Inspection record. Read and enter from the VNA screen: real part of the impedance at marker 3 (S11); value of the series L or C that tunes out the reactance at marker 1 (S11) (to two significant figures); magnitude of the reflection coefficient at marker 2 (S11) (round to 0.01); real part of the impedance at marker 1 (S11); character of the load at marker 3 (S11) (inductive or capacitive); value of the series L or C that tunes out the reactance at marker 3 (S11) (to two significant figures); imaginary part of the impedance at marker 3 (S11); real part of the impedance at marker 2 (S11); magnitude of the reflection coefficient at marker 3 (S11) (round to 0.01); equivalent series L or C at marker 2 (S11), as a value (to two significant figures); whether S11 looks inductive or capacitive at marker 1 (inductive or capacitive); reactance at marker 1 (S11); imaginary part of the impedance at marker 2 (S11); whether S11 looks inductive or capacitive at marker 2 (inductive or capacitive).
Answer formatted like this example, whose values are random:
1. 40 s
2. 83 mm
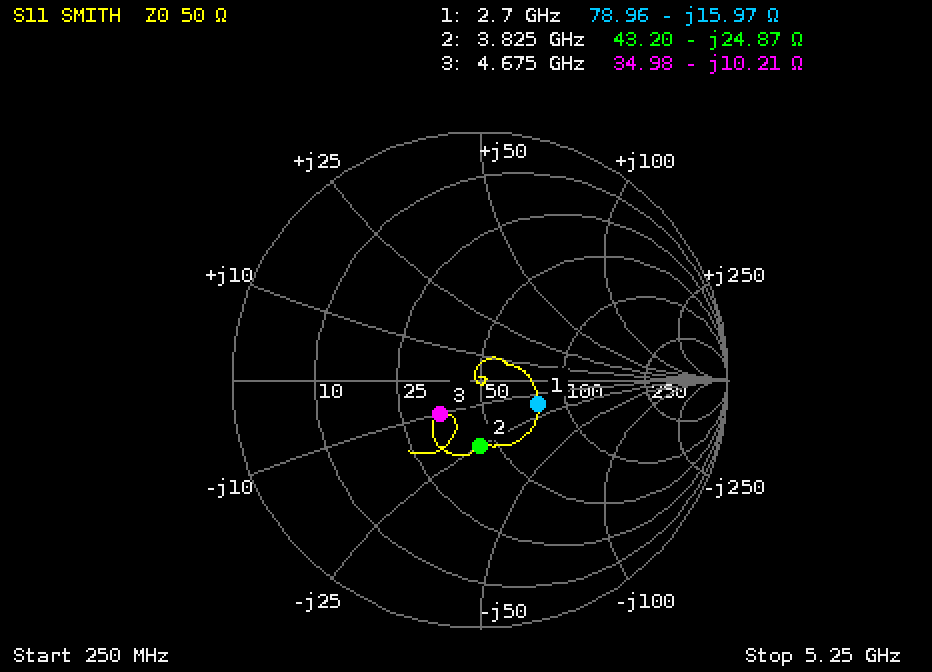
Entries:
1. 34.98 Ω
2. 940 pH
3. 0.27
4. 78.96 Ω
5. capacitive
6. 350 pH
7. -10.21 Ω
8. 43.20 Ω
9. 0.21
10. 1.7 pF
11. capacitive
12. -15.97 Ω
13. -24.87 Ω
14. capacitive
